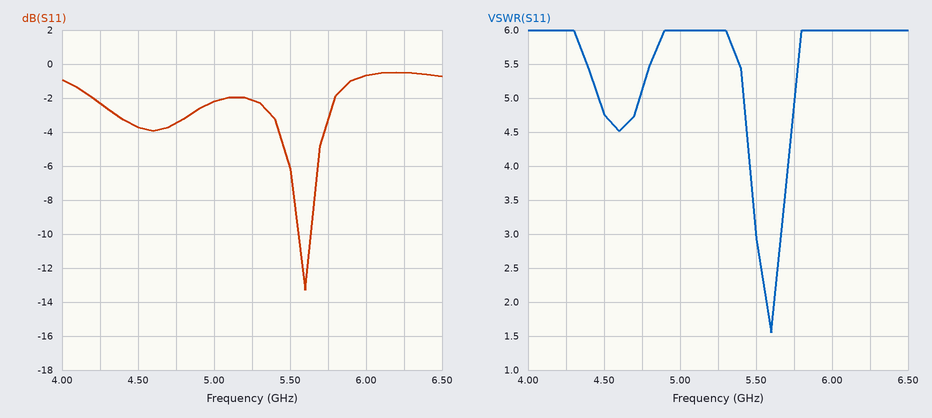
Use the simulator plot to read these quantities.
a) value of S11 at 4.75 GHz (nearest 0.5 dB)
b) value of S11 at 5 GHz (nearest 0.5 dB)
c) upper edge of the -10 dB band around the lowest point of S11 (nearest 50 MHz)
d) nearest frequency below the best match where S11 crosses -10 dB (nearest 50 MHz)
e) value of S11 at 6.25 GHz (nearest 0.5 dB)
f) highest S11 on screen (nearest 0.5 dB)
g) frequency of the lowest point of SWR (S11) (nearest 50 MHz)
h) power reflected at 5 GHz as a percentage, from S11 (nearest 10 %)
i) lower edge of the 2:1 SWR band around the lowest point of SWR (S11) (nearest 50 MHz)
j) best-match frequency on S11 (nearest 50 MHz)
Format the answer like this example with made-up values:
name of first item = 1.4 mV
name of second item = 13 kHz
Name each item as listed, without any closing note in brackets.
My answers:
value of S11 at 4.75 GHz = -3.5 dB
value of S11 at 5 GHz = -2.0 dB
upper edge of the -10 dB band around the lowest point of S11 = 5.65 GHz
nearest frequency below the best match where S11 crosses -10 dB = 5.55 GHz
value of S11 at 6.25 GHz = -0.5 dB
highest S11 on screen = -0.5 dB
frequency of the lowest point of SWR (S11) = 5.60 GHz
power reflected at 5 GHz as a percentage, from S11 = 60 %
lower edge of the 2:1 SWR band around the lowest point of SWR (S11) = 5.55 GHz
best-match frequency on S11 = 5.60 GHz
